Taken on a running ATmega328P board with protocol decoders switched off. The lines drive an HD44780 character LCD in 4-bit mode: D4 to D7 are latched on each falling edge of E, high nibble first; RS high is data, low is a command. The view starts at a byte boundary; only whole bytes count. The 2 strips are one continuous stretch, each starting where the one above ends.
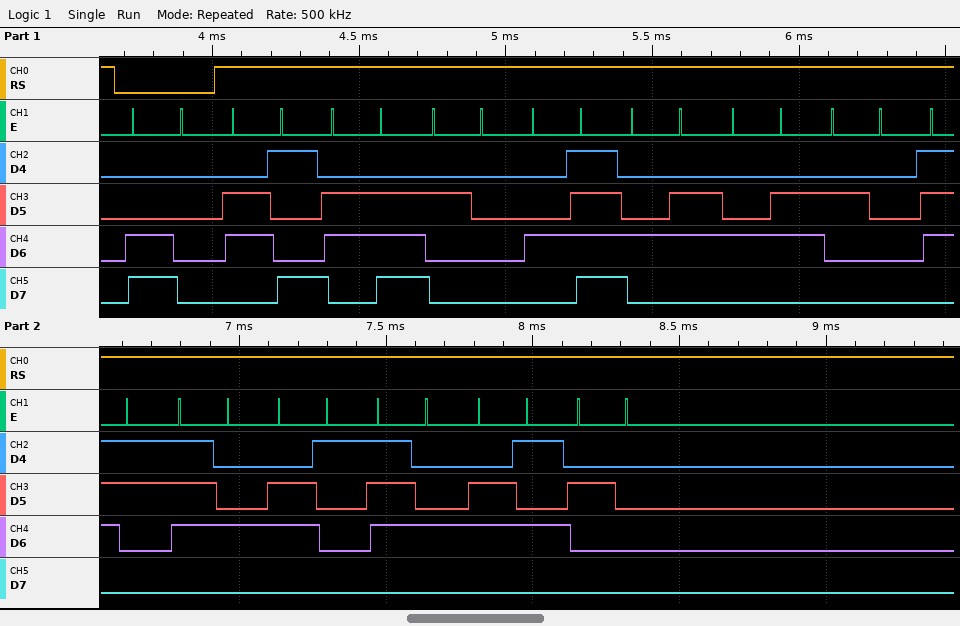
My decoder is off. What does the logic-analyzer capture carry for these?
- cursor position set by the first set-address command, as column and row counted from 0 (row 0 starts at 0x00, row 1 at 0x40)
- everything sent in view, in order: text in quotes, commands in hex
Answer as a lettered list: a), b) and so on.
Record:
a) column 0, row 1
b) 0xC0 "in OFF state "
